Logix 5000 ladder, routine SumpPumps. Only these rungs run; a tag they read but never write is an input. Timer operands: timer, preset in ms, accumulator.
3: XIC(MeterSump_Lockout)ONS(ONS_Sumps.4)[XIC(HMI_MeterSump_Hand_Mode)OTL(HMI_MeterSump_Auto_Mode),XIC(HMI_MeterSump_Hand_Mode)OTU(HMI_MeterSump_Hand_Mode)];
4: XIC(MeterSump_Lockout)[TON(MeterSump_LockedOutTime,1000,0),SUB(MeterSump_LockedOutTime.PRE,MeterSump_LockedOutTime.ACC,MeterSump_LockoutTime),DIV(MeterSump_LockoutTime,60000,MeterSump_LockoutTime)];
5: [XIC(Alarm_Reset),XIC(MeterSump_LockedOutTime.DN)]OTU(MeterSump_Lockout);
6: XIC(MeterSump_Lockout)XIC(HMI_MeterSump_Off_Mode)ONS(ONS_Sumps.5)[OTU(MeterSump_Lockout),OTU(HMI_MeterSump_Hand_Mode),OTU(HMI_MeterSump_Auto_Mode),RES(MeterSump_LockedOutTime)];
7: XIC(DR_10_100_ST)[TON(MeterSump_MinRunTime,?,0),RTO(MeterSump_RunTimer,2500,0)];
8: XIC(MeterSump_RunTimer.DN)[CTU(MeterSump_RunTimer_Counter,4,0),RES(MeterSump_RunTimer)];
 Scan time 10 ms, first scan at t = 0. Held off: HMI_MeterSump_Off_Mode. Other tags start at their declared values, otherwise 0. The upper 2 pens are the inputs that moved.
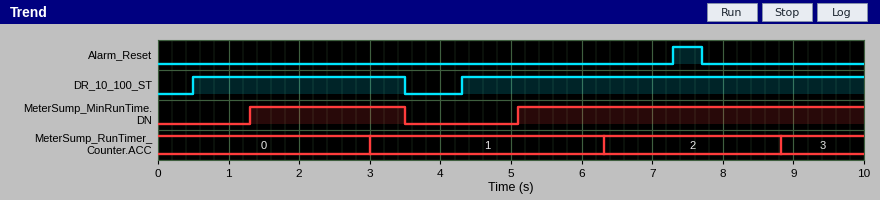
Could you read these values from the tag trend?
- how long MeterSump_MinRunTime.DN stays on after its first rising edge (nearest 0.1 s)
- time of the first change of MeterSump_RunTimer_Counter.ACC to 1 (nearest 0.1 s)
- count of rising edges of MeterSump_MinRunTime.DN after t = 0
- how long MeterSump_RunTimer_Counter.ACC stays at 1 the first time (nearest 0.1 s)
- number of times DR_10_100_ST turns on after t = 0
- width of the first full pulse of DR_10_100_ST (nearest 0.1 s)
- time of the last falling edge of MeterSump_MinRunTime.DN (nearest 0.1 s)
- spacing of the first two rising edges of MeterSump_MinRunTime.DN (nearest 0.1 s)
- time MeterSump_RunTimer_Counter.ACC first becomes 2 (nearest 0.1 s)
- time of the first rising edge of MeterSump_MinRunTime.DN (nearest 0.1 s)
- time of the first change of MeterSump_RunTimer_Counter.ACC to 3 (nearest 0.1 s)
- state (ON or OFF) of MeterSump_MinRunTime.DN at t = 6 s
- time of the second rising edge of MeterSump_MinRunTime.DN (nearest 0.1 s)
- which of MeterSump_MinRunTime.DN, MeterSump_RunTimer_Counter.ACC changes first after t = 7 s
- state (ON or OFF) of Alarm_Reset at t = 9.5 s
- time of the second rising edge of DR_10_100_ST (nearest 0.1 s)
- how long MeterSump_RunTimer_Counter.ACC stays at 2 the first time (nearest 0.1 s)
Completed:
2.2 s
3.0 s
2
3.3 s
2
3.0 s
3.5 s
3.8 s
6.3 s
1.3 s
8.8 s
ON
5.1 s
MeterSump_RunTimer_Counter.ACC
OFF
4.3 s
2.5 s
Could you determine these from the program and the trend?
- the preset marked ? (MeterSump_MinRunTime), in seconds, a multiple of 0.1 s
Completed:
0.8 s
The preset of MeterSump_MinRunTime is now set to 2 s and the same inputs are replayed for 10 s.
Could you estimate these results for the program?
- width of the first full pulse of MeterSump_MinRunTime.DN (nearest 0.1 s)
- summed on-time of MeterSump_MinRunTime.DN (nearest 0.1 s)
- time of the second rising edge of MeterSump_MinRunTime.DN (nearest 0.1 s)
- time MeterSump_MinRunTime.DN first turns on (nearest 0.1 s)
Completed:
1.0 s
4.7 s
6.3 s
2.5 s
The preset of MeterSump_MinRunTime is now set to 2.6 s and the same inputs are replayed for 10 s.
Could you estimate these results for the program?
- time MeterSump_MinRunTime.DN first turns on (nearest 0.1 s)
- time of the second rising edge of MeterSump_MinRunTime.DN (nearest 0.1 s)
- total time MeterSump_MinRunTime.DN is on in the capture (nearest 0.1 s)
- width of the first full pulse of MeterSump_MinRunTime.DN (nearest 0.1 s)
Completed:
3.1 s
6.9 s
3.5 s
0.4 s
